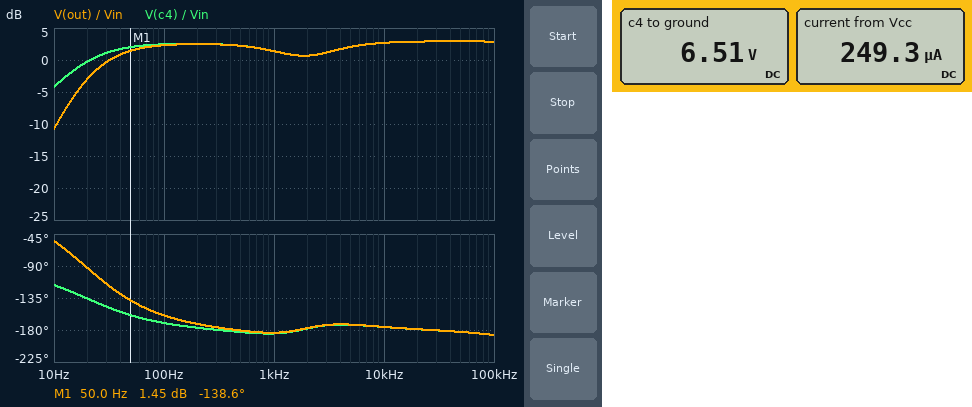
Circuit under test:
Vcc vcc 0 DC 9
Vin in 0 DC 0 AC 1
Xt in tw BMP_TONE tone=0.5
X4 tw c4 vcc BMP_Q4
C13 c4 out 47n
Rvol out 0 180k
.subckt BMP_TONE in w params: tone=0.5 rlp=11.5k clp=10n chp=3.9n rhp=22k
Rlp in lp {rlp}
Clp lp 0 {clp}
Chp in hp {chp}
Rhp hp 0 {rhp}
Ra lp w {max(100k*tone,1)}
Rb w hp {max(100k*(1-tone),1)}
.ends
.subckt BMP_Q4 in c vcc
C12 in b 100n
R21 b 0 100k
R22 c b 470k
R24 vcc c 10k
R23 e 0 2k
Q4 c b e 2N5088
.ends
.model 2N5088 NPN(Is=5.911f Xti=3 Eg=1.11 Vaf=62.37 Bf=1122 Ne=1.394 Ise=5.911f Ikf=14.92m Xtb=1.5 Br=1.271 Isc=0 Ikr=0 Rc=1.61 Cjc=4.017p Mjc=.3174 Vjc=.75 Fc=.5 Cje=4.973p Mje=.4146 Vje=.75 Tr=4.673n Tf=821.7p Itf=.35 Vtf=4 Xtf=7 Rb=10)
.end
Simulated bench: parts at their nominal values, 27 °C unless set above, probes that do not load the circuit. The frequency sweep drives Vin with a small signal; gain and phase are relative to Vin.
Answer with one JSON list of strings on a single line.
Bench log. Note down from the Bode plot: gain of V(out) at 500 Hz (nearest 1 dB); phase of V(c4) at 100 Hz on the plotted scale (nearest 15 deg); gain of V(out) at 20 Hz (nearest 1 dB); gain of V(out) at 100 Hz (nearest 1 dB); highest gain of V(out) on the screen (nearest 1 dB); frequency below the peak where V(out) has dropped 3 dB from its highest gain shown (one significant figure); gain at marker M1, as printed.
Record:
["2 dB", "-165 deg", "-3 dB", "2 dB", "3 dB", "30 Hz", "1.45 dB"]
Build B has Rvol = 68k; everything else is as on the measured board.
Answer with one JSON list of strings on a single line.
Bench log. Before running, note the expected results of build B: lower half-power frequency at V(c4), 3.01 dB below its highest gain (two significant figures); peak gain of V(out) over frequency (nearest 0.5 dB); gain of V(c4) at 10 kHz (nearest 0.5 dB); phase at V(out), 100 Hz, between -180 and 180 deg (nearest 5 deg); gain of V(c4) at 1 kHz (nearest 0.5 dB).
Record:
["18 Hz", "2.5 dB", "2.0 dB", "-145 deg", "1.0 dB"]
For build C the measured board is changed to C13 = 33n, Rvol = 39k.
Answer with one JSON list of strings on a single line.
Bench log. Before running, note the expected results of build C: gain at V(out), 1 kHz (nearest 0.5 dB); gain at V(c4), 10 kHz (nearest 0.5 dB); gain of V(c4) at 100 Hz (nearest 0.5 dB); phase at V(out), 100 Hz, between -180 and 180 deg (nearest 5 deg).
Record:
["0 dB", "1.5 dB", "2.0 dB", "-125 deg"]
